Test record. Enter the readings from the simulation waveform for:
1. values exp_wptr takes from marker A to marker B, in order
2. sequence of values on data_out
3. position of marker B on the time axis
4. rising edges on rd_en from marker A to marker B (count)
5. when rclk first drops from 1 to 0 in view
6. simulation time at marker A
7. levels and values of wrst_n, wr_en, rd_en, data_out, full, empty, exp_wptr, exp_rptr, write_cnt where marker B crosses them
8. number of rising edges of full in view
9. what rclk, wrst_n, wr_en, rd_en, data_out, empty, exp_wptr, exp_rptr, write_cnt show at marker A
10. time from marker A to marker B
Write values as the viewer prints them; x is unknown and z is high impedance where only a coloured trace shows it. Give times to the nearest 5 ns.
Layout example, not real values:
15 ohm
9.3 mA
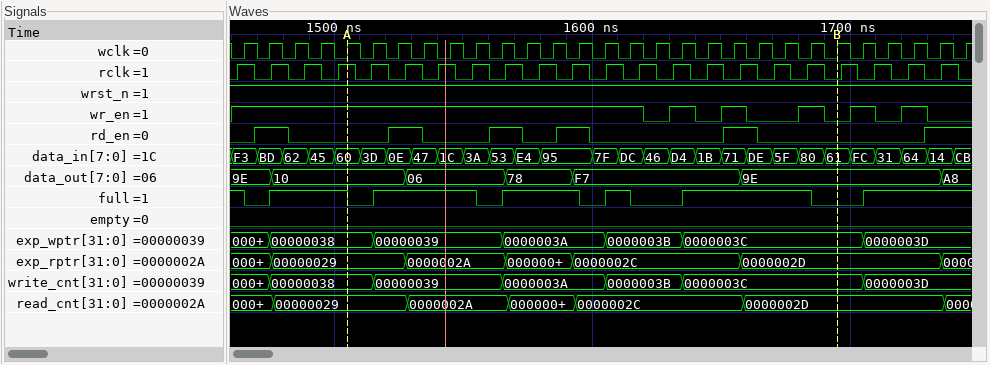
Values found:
00000038, 00000039, 0000003A, 0000003B, 0000003C
9E, 10, 06, 78, F7, 9E, A8
1695 ns
4
1470 ns
1505 ns
wrst_n=1, wr_en=0, rd_en=0, data_out=9E, full=0, empty=0, exp_wptr=0000003C, exp_rptr=0000002D, write_cnt=0000003C
6
rclk=1, wrst_n=1, wr_en=1, rd_en=0, data_out=10, empty=0, exp_wptr=00000038, exp_rptr=00000029, write_cnt=00000038
190 ns
